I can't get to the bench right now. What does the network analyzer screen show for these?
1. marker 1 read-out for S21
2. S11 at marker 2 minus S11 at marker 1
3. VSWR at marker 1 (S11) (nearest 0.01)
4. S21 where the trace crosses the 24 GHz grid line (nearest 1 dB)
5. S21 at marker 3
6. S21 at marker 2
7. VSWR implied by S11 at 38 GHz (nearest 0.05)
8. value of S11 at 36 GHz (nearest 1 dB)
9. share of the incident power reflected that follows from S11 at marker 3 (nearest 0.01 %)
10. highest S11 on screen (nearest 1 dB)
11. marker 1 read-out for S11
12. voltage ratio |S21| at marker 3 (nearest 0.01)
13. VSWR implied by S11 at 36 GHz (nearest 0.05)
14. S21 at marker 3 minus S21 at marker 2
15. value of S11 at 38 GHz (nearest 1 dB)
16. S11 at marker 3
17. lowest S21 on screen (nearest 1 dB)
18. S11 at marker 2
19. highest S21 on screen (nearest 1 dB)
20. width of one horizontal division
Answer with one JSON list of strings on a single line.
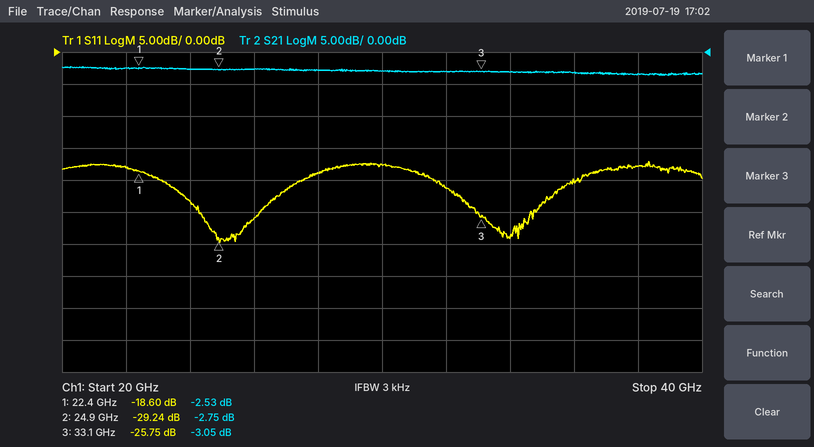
["-2.53 dB", "-10.64 dB", "1.27", "-3 dB", "-3.05 dB", "-2.75 dB", "1.30", "-20 dB", "0.27 %", "-17 dB", "-18.60 dB", "0.70", "1.20", "-0.30 dB", "-18 dB", "-25.75 dB", "-4 dB", "-29.24 dB", "-2 dB", "2 GHz"]
